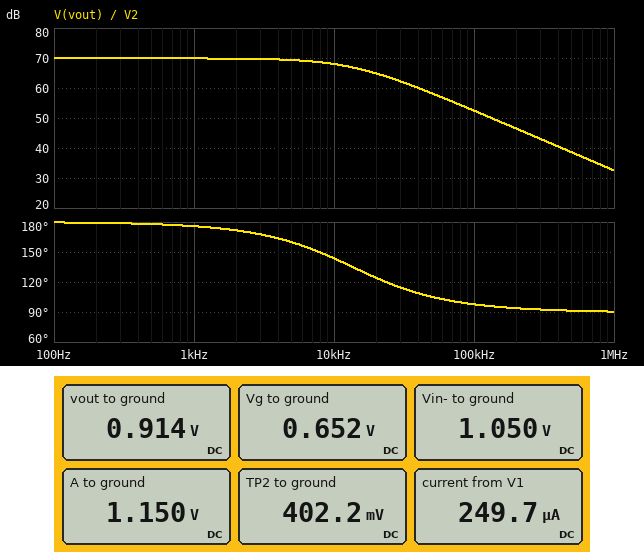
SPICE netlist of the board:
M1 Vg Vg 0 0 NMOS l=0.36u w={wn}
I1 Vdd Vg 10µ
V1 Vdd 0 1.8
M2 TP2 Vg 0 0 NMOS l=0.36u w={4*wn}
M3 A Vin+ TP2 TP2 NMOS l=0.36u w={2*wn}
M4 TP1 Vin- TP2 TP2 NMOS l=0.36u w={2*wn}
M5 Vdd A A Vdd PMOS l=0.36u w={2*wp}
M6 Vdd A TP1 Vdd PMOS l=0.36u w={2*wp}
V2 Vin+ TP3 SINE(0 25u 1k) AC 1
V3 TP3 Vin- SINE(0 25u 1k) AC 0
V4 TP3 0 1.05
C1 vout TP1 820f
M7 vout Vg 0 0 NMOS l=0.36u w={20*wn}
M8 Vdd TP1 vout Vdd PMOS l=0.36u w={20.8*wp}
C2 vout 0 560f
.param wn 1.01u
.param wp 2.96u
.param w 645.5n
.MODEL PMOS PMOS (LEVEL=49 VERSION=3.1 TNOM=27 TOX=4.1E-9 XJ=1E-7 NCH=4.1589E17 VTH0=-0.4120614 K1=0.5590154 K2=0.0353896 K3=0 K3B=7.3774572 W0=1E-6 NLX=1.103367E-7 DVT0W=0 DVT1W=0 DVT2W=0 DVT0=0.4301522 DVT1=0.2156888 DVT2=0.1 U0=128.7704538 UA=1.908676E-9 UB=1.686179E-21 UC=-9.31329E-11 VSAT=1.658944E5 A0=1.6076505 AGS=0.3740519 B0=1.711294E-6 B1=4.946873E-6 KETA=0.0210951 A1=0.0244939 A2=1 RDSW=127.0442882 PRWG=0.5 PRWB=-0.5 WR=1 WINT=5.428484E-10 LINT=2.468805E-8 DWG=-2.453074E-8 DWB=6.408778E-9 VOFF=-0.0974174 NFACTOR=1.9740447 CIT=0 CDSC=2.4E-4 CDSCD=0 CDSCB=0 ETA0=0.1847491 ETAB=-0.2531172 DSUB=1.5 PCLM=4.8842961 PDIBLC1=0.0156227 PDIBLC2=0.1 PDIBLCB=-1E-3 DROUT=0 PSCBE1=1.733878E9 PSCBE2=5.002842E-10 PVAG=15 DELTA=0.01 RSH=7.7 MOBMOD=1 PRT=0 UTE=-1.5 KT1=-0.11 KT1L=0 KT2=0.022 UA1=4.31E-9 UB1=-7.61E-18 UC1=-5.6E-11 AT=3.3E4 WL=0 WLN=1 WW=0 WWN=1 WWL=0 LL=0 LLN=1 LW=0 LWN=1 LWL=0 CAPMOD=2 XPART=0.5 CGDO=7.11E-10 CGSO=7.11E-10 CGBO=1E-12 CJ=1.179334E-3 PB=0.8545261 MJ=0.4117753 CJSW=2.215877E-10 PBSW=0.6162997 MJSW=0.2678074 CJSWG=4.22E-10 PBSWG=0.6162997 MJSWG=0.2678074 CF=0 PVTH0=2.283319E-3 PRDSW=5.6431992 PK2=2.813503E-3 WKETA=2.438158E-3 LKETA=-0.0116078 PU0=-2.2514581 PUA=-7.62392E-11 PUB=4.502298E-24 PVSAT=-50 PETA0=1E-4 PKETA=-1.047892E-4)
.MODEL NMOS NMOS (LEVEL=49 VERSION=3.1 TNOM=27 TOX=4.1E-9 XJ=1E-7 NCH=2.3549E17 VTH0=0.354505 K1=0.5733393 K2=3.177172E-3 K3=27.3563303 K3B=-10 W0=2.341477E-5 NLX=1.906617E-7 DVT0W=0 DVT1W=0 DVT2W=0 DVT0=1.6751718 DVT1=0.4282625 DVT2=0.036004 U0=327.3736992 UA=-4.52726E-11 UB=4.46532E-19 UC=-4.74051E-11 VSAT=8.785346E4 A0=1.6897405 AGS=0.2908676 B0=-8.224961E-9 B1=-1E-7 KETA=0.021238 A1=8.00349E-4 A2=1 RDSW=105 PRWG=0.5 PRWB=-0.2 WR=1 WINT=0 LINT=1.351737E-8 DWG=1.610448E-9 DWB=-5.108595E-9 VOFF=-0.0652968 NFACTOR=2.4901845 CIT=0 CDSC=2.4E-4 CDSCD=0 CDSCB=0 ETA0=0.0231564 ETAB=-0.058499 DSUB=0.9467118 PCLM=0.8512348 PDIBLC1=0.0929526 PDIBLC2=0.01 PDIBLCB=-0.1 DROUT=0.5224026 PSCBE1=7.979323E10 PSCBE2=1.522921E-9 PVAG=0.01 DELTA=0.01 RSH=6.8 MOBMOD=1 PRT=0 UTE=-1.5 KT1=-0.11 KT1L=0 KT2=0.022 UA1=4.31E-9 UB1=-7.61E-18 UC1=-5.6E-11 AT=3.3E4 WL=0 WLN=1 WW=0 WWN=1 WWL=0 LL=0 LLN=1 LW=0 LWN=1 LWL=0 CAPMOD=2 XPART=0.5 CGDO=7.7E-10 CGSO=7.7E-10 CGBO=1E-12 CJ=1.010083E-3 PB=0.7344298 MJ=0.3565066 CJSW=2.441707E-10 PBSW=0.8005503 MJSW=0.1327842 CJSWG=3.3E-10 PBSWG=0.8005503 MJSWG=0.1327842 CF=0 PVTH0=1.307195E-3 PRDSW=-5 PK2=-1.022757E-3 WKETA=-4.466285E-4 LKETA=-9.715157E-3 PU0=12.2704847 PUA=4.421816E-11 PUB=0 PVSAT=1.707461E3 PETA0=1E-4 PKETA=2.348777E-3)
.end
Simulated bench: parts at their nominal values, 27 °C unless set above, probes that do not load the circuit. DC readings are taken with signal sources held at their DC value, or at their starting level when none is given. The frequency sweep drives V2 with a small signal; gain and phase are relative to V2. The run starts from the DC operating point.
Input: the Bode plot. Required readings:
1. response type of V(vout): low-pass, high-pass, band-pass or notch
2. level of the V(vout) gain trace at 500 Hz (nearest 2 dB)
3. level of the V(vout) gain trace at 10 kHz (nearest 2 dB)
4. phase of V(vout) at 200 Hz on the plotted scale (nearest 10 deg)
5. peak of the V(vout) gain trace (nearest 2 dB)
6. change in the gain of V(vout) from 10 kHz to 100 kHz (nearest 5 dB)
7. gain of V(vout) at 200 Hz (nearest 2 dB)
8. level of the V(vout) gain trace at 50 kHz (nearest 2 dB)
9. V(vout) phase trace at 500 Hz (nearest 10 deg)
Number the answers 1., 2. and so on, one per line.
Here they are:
1. low-pass
2. 70 dB
3. 68 dB
4. 180 deg
5. 70 dB
6. -15 dB
7. 70 dB
8. 58 dB
9. 180 deg
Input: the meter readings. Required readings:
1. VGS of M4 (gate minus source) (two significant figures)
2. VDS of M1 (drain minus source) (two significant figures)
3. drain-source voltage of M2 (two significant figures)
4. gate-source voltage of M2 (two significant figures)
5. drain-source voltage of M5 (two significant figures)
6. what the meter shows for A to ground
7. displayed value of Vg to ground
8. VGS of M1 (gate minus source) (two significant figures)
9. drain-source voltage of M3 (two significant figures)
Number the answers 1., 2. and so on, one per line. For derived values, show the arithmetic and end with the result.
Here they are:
1. 1.05 V - 402.2 mV = 650 mV
2. 652 mV = 650 mV
3. 402.2 mV = 400 mV
4. 652 mV = 650 mV
5. 1.8 V - 1.15 V = 650 mV
6. 1.150 V
7. 0.652 V
8. 652 mV = 650 mV
9. 1.15 V - 402.2 mV = 750 mV
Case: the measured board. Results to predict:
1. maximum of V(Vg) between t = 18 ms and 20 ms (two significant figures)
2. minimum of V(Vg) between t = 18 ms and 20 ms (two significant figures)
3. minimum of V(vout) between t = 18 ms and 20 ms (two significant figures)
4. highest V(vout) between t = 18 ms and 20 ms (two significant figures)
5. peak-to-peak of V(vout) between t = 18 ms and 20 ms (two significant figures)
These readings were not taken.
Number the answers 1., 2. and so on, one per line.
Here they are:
1. 650 mV
2. 650 mV
3. 760 mV
4. 1.1 V
5. 310 mV
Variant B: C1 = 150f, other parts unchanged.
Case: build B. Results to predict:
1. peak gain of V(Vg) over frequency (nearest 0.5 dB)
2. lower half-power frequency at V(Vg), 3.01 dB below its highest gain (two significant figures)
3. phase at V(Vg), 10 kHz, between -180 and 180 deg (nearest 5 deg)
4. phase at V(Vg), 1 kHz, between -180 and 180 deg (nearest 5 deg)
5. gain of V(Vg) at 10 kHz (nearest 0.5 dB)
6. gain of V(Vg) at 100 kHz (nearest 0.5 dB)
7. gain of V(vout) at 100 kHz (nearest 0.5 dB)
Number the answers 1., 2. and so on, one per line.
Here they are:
1. -17.0 dB
2. 59 kHz
3. -100 deg
4. -90 deg
5. -32.5 dB
6. -18.0 dB
7. 64.0 dB
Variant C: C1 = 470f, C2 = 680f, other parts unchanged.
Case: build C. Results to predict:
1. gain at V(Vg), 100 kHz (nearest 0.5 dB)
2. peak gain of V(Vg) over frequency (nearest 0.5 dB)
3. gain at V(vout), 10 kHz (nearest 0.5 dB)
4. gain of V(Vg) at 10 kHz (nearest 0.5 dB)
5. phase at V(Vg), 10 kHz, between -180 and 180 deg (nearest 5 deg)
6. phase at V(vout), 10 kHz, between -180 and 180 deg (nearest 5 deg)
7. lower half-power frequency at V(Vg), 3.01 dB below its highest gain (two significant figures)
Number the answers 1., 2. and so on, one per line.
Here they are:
1. -25.5 dB
2. -25.0 dB
3. 69.0 dB
4. -33.0 dB
5. -115 deg
6. 155 deg
7. 23 kHz
